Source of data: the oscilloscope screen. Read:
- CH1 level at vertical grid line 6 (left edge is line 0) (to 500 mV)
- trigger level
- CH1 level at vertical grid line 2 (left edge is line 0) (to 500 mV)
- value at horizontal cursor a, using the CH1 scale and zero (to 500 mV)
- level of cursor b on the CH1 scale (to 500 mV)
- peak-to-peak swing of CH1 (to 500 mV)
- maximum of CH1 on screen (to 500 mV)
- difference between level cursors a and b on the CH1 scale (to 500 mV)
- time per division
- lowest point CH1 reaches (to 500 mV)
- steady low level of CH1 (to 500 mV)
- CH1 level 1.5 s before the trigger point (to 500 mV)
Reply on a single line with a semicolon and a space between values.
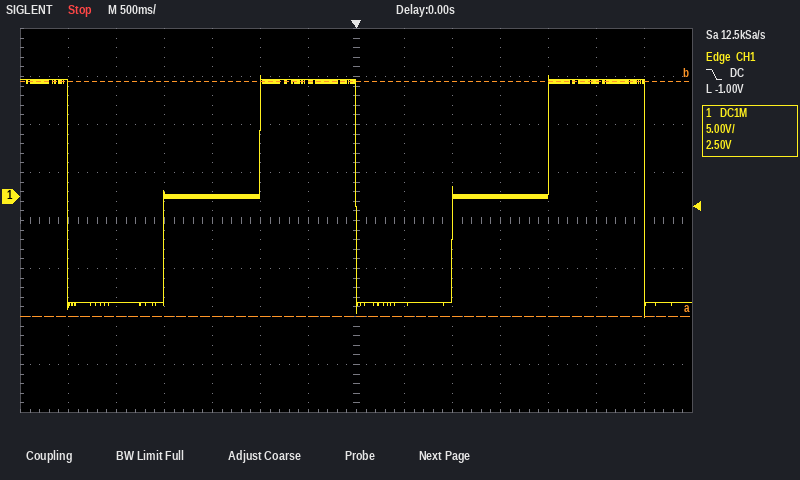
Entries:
12.0 V; -1.00 V; -11.0 V; -12.5 V; 12.0 V; 25.0 V; 12.5 V; 24.5 V; 500 ms; -12.5 V; -11.0 V; 0.0 V
